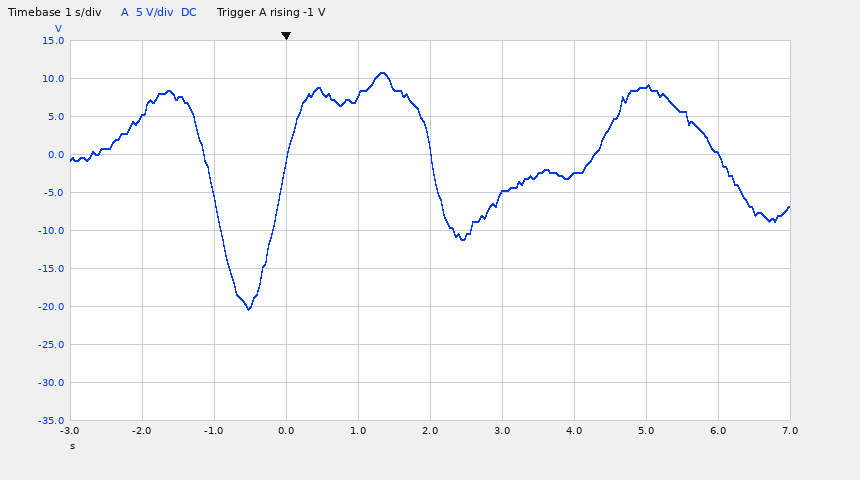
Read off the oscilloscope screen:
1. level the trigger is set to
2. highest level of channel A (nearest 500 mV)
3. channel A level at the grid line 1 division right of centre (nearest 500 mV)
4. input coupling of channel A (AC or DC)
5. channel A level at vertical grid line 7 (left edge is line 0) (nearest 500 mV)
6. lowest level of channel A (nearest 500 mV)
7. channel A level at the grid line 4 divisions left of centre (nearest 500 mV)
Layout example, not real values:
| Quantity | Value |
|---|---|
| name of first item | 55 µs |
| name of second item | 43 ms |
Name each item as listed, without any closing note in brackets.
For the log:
| Quantity | Value |
|---|---|
| level the trigger is set to | -1 V |
| highest level of channel A | 11.0 V |
| channel A level at the grid line 1 division right of centre | -5.0 V |
| input coupling of channel A | DC |
| channel A level at vertical grid line 7 (left edge is line 0) | -2.5 V |
| lowest level of channel A | -20.5 V |
| channel A level at the grid line 4 divisions left of centre | 5.0 V |
